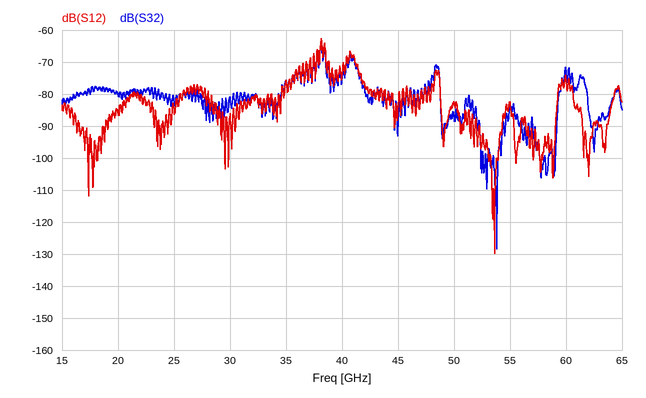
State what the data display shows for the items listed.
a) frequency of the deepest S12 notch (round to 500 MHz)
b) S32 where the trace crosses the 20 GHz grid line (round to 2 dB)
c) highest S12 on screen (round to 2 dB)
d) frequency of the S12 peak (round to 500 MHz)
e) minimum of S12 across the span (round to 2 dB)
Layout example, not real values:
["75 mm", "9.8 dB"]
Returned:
["53.5 GHz", "-80 dB", "-62 dB", "38.0 GHz", "-130 dB"]
